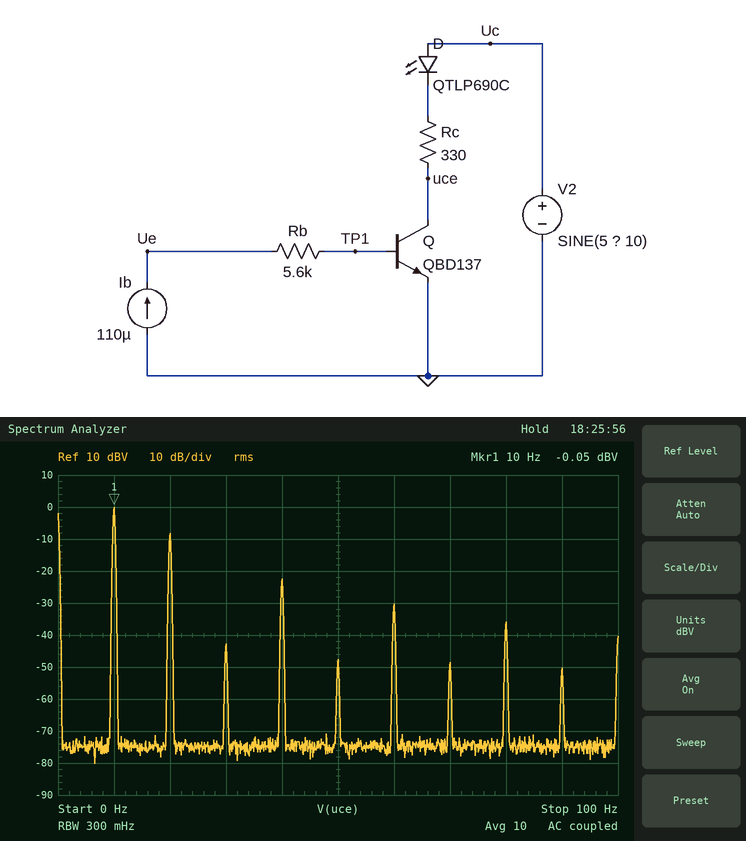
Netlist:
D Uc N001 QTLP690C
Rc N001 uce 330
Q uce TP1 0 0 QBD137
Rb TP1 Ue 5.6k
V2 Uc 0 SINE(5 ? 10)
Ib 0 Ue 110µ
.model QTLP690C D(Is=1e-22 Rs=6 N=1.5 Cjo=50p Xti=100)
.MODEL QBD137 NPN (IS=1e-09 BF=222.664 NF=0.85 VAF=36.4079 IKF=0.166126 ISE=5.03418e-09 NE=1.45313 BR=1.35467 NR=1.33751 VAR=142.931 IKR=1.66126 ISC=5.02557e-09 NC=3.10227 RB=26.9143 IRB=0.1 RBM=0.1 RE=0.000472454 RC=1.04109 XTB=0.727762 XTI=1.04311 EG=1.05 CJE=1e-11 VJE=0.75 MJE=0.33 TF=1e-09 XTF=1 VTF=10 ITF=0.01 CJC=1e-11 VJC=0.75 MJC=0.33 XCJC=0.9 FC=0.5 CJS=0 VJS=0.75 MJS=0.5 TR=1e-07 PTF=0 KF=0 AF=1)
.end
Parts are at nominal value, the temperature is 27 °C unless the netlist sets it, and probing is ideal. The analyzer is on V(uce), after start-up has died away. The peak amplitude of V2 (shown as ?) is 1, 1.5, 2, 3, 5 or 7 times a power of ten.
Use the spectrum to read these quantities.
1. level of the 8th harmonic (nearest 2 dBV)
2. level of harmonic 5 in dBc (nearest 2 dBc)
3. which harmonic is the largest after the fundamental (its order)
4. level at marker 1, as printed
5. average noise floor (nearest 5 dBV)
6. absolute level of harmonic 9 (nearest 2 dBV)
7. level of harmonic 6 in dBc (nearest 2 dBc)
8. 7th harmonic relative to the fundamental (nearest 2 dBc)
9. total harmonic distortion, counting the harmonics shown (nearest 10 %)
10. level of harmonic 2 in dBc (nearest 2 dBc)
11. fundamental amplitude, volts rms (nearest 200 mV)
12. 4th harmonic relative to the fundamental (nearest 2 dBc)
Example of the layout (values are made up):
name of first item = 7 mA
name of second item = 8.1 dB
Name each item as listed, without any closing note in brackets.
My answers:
level of the 8th harmonic = -36 dBV
level of harmonic 5 in dBc = -48 dBc
which harmonic is the largest after the fundamental = 2
level at marker 1, as printed = -0.05 dBV
average noise floor = -75 dBV
absolute level of harmonic 9 = -50 dBV
level of harmonic 6 in dBc = -30 dBc
7th harmonic relative to the fundamental = -48 dBc
total harmonic distortion, counting the harmonics shown = 40 %
level of harmonic 2 in dBc = -8 dBc
fundamental amplitude, volts rms = 1.0 V
4th harmonic relative to the fundamental = -22 dBc
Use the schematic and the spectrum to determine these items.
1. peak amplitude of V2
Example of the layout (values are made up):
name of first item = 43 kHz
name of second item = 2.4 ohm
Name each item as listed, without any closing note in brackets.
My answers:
peak amplitude of V2 = 3 V
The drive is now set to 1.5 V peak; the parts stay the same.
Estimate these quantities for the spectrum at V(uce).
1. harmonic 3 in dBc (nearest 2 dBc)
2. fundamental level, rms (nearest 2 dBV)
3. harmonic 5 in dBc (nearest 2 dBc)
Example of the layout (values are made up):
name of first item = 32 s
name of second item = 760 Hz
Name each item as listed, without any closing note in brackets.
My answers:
harmonic 3 in dBc = -36 dBc
fundamental level, rms = -6 dBV
harmonic 5 in dBc = -38 dBc
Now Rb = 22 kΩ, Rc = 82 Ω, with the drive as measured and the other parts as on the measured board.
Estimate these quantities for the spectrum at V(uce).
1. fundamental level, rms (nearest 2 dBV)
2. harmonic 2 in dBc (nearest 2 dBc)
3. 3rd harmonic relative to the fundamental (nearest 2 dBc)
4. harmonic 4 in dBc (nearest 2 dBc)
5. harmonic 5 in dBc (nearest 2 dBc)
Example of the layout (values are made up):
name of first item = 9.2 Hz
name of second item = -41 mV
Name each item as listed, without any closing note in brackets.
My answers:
fundamental level, rms = 6 dBV
harmonic 2 in dBc = -26 dBc
3rd harmonic relative to the fundamental = -28 dBc
harmonic 4 in dBc = -32 dBc
harmonic 5 in dBc = -38 dBc
